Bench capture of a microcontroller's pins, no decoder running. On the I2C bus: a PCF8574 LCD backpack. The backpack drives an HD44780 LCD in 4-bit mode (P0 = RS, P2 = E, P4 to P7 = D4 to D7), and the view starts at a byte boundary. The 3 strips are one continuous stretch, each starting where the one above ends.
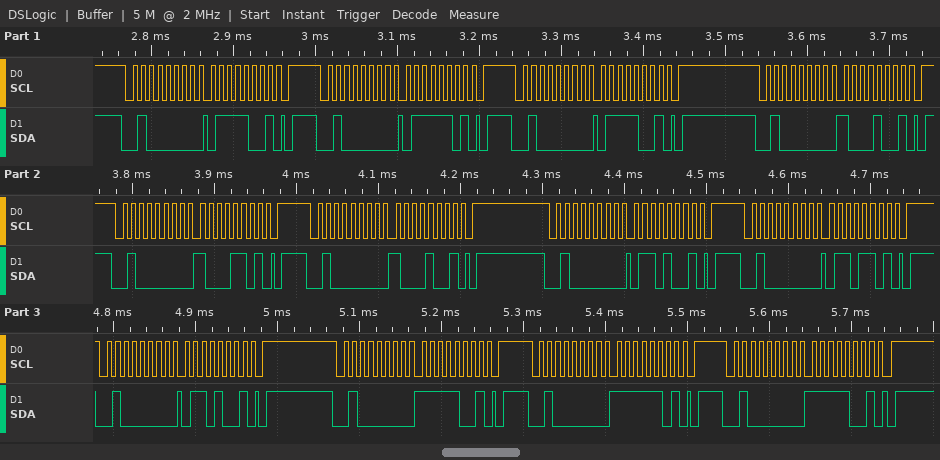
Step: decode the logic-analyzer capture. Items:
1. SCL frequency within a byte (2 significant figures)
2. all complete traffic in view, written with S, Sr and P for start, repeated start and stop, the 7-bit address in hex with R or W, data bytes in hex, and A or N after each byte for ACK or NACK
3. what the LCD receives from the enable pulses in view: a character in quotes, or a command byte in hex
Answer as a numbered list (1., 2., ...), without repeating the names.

1. 100 kHz
2. S 20W A 79 A P S 20W A 7D A P S 20W A 79 A P S 20W A 89 A P S 20W A 8D A P S 20W A 89 A P S 20W A 69 A P S 20W A 6D A P S 20W A 69 A P S 20W A F9 A P S 20W A FD A P S 20W A F9 A P
3. 'x' 'o'
